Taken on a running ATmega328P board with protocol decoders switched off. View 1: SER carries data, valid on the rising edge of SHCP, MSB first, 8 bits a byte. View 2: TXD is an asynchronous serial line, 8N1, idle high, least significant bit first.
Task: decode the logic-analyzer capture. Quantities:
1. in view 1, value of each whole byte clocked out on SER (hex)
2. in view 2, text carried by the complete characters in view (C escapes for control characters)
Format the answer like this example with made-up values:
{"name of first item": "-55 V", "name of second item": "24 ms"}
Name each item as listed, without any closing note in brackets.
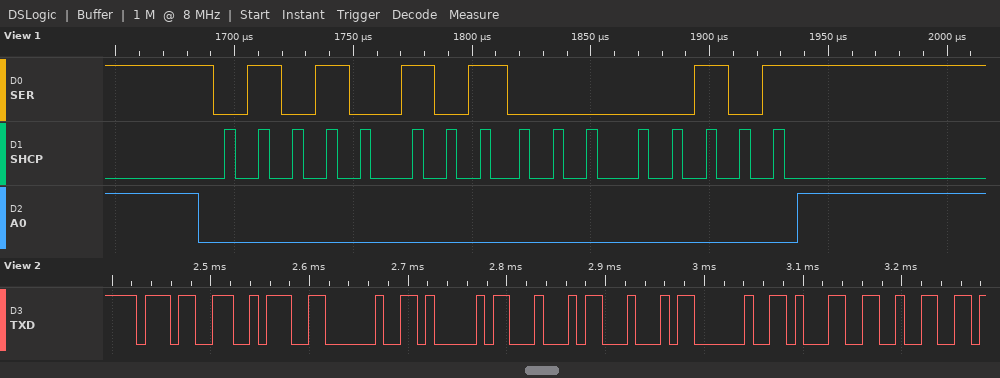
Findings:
{"in view 1, value of each whole byte clocked out on SER": "55 05", "in view 2, text carried by the complete characters in view": "\"7: ADD 12\""}
